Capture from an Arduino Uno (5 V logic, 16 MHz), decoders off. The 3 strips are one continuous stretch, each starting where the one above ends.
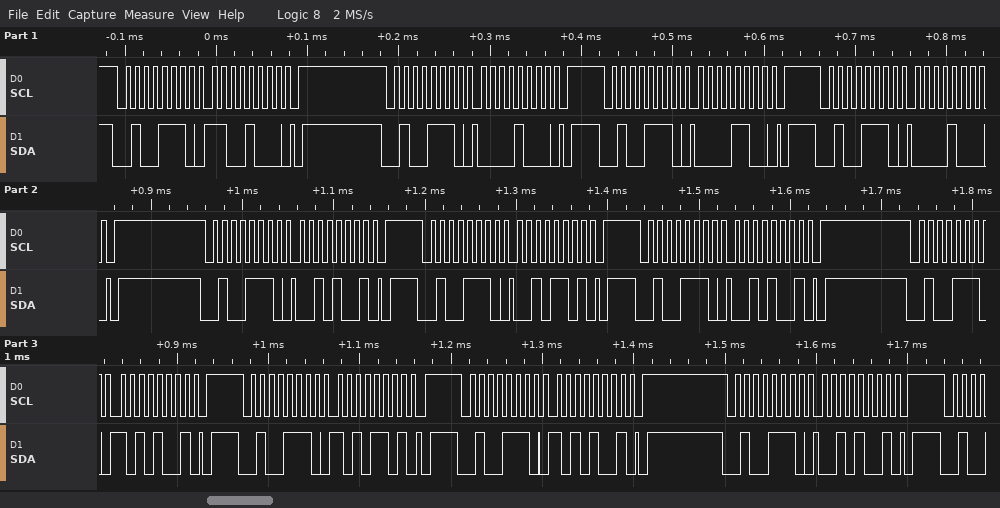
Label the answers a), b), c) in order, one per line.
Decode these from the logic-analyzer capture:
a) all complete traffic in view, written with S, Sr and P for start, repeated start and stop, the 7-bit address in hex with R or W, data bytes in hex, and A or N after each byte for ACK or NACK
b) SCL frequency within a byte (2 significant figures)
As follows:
a) S 27W A C8 A P S 27W A 08 A P S 27W A 0C A P S 27W A 08 A P S 27W A 29 A P S 27W A 2D A P S 27W A 29 A P S 27W A A9 A P S 27W A AD A P S 27W A A9 A P S 27W A 29 A P
b) 100 kHz
